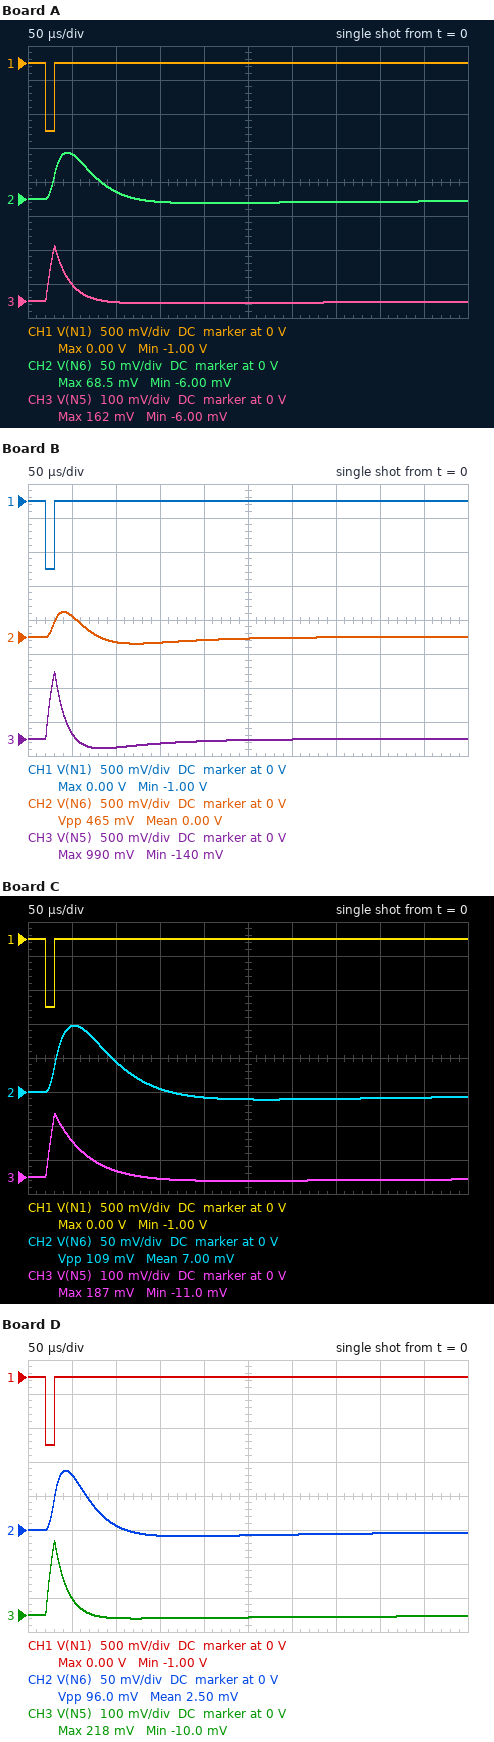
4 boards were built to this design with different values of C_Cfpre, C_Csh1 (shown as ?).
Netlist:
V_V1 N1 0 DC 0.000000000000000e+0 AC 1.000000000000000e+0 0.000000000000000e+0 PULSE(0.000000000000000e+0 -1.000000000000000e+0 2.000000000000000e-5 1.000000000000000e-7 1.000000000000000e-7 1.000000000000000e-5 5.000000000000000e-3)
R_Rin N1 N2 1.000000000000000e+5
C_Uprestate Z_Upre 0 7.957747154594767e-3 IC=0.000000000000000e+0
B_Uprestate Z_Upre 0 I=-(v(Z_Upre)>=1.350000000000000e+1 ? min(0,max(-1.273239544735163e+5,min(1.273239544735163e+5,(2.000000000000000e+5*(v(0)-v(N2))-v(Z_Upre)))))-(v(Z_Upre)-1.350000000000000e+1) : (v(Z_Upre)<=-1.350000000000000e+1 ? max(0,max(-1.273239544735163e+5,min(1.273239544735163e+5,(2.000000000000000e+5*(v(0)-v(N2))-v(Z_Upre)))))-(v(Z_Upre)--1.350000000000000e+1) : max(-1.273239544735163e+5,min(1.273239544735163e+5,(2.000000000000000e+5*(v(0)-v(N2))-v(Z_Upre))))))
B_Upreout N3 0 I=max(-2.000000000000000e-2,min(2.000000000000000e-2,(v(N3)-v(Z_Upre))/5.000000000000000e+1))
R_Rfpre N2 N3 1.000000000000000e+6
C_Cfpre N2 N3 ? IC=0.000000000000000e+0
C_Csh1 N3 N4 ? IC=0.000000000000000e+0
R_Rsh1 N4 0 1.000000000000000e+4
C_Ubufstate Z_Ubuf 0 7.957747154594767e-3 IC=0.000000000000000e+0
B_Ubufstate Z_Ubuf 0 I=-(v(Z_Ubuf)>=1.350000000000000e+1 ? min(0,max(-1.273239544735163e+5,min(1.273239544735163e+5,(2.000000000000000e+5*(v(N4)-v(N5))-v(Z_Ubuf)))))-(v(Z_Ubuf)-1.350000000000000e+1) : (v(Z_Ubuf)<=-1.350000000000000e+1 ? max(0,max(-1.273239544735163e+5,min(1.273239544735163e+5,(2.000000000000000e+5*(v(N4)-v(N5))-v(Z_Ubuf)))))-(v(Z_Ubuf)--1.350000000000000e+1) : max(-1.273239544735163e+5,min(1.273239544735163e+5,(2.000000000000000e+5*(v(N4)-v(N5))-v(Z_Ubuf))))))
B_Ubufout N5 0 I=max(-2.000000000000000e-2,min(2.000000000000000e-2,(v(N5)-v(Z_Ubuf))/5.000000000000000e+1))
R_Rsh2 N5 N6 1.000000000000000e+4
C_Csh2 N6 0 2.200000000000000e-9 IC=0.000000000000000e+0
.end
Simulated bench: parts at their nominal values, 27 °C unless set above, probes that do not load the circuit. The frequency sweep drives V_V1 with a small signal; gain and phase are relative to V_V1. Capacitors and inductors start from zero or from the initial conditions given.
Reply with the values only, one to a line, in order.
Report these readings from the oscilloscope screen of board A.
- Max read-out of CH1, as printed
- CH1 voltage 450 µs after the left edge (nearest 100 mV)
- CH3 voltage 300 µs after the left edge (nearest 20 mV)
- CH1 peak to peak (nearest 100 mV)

0.00 V
0 V
0 V
1.0 V
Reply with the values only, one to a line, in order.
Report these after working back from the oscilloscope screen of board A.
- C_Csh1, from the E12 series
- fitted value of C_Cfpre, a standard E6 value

1.8 nF
470 pF
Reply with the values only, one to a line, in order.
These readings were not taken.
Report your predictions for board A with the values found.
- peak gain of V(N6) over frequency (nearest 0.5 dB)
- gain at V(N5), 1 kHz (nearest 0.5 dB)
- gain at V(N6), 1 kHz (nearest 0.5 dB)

-9.0 dB
-9.0 dB
-9.0 dB
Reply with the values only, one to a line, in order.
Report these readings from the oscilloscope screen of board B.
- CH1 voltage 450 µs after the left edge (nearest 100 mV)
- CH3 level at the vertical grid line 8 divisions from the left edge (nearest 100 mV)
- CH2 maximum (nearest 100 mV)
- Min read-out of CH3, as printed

0 V
0 V
400 mV
-140 mV
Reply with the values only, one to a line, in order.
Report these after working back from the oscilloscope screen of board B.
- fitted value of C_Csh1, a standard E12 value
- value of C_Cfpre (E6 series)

1.5 nF
68 pF
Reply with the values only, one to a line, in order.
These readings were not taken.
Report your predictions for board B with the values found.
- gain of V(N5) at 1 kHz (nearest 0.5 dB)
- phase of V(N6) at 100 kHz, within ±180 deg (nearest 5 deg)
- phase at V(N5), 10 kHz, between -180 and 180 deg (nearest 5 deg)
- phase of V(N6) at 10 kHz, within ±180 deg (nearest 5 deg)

-1.5 dB
10 deg
150 deg
95 deg
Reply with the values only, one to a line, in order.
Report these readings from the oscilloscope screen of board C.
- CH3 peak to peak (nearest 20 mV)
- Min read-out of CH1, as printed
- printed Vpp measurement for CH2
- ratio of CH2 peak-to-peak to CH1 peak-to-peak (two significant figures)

200 mV
-1.00 V
109 mV
0.11
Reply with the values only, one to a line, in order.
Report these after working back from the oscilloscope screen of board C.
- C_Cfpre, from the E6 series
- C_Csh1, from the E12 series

470 pF
3.9 nF
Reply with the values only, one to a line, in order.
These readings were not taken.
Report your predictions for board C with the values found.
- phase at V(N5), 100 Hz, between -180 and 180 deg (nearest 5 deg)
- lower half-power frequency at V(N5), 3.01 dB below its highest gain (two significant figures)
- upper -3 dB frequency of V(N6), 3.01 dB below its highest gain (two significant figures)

-110 deg
290 Hz
3.8 kHz
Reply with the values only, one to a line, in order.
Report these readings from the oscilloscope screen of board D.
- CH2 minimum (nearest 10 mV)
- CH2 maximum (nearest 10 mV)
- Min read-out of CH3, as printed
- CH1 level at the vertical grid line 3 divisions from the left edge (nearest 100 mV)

-10 mV
90 mV
-10.0 mV
0 V
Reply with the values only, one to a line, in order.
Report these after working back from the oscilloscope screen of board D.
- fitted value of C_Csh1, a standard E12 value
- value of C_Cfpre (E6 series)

1.5 nF
330 pF
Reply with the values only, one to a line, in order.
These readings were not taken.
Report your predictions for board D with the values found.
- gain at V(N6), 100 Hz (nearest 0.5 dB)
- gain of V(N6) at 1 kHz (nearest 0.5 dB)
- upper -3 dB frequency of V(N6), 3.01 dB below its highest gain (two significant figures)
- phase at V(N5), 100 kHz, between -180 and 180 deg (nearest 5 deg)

-20.5 dB
-8.0 dB
6.2 kHz
95 deg
